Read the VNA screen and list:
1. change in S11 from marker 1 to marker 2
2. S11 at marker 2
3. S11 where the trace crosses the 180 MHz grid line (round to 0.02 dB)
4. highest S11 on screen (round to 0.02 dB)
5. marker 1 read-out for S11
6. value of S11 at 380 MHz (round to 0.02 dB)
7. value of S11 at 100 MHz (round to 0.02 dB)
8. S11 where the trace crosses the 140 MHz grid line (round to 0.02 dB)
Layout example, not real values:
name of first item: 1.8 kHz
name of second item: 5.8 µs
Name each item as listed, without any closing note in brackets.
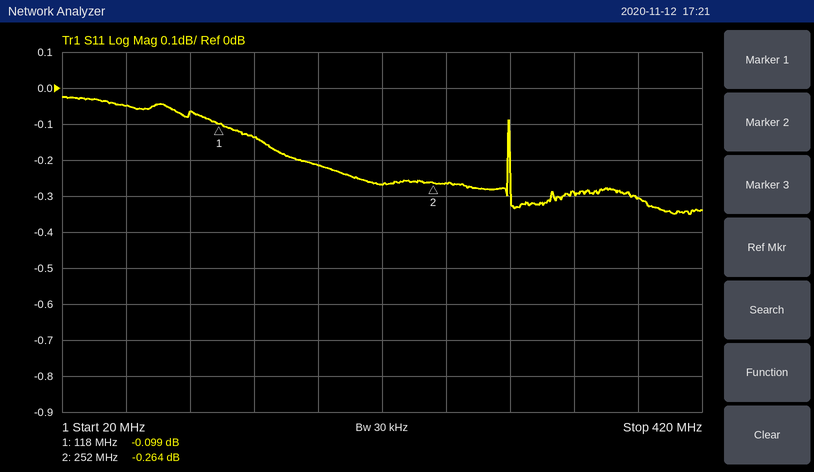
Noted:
change in S11 from marker 1 to marker 2: -0.165 dB
S11 at marker 2: -0.264 dB
S11 where the trace crosses the 180 MHz grid line: -0.22 dB
highest S11 on screen: -0.02 dB
marker 1 read-out for S11: -0.099 dB
value of S11 at 380 MHz: -0.30 dB
value of S11 at 100 MHz: -0.06 dB
S11 where the trace crosses the 140 MHz grid line: -0.14 dB
